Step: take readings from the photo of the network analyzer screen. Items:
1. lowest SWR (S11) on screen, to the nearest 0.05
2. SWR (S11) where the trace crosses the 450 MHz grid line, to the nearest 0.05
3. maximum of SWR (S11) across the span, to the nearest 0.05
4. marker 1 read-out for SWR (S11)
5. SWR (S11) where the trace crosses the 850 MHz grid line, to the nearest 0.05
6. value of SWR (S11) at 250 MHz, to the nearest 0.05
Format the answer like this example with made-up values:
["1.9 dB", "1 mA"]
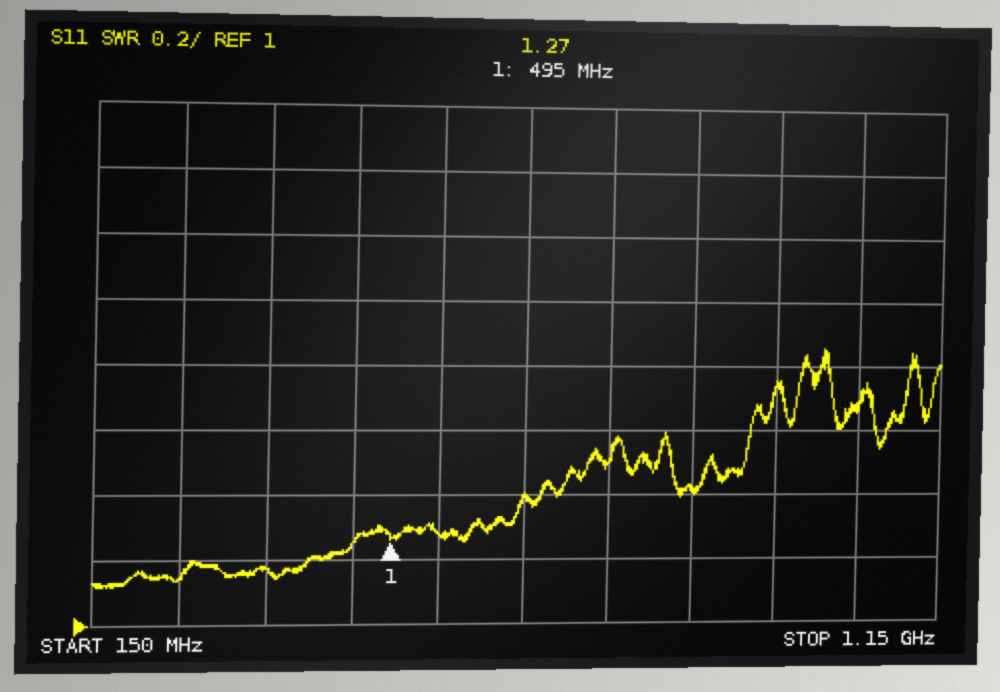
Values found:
["1.10", "1.25", "1.85", "1.27", "1.40", "1.15"]
